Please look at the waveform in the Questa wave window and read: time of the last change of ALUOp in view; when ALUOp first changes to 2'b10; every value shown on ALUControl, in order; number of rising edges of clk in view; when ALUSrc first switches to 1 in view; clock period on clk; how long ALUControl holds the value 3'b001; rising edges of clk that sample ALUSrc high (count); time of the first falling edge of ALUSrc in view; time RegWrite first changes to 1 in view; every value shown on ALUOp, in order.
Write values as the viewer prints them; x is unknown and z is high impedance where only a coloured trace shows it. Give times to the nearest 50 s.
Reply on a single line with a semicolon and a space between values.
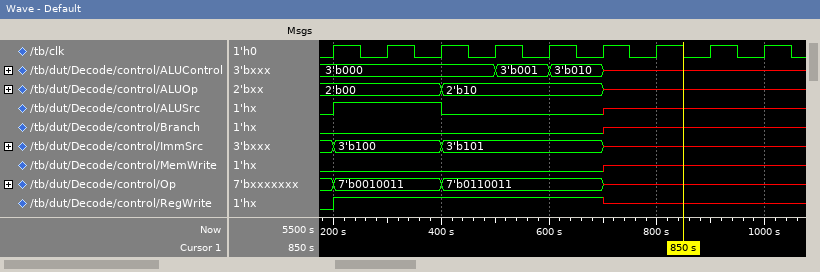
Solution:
700 s; 400 s; 3'b000, 3'b001, 3'b010, x; 9; 200 s; 100 s; 100 s; 2; 400 s; 200 s; 2'b00, 2'b10, x
